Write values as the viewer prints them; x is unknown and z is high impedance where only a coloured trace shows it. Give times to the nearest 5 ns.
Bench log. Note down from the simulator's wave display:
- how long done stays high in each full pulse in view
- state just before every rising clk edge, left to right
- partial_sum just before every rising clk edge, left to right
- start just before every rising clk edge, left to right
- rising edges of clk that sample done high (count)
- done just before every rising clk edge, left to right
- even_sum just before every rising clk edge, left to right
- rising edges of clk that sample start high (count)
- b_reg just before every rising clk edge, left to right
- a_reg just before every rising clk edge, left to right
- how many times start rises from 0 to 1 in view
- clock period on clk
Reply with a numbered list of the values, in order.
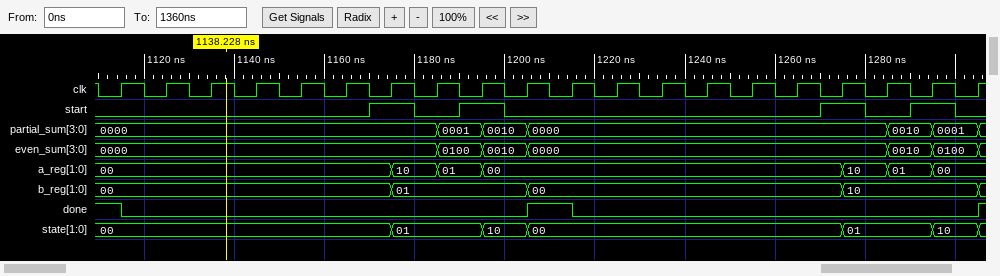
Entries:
1. 10 ns
2. 00, 00, 00, 00, 00, 00, 00, 01, 01, 10, 00, 00, 00, 00, 00, 00, 00, 01, 01, 10
3. 0000, 0000, 0000, 0000, 0000, 0000, 0000, 0000, 0001, 0010, 0000, 0000, 0000, 0000, 0000, 0000, 0000, 0000, 0010, 0001
4. 0 0 0 0 0 0 1 0 1 0 0 0 0 0 0 0 1 0 1 0
5. 2
6. 1 0 0 0 0 0 0 0 0 0 1 0 0 0 0 0 0 0 0 0
7. 0000, 0000, 0000, 0000, 0000, 0000, 0000, 0000, 0100, 0010, 0000, 0000, 0000, 0000, 0000, 0000, 0000, 0000, 0010, 0100
8. 4
9. 00, 00, 00, 00, 00, 00, 00, 01, 01, 01, 00, 00, 00, 00, 00, 00, 00, 10, 10, 10
10. 00, 00, 00, 00, 00, 00, 00, 10, 01, 00, 00, 00, 00, 00, 00, 00, 00, 10, 01, 00
11. 4
12. 10 ns
